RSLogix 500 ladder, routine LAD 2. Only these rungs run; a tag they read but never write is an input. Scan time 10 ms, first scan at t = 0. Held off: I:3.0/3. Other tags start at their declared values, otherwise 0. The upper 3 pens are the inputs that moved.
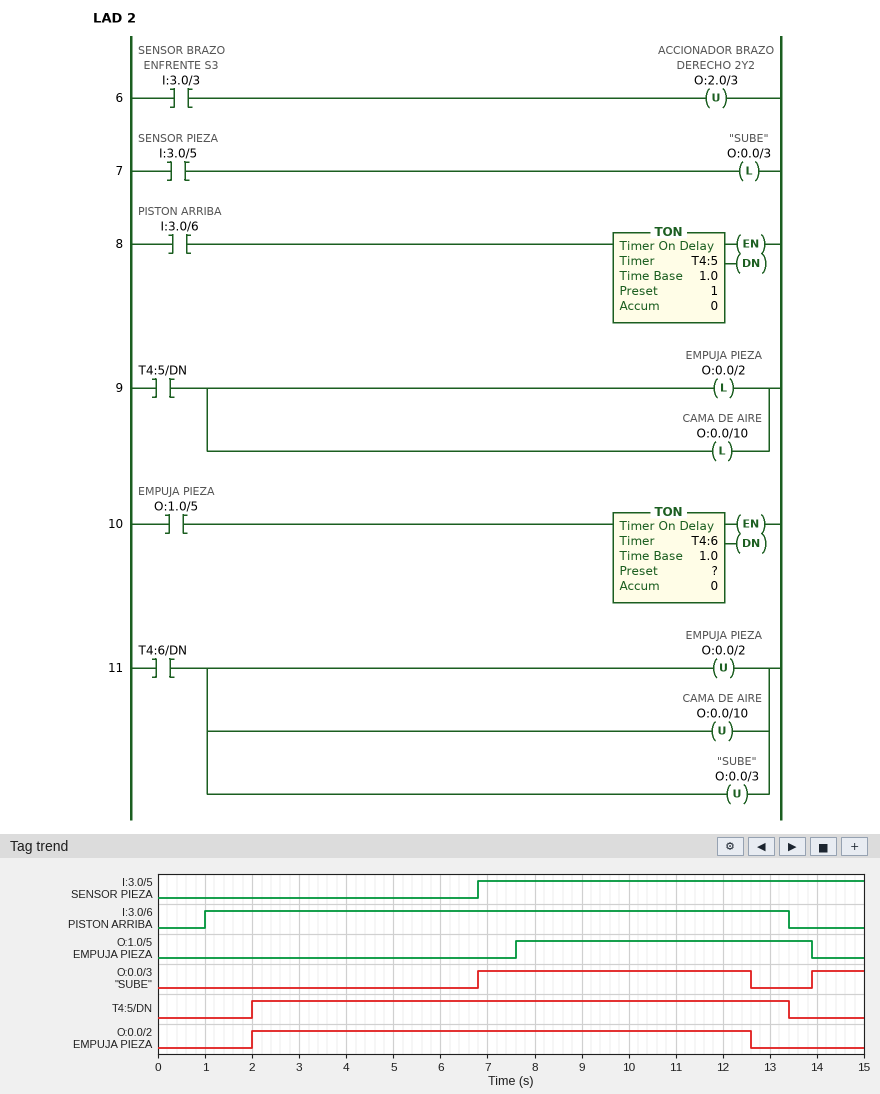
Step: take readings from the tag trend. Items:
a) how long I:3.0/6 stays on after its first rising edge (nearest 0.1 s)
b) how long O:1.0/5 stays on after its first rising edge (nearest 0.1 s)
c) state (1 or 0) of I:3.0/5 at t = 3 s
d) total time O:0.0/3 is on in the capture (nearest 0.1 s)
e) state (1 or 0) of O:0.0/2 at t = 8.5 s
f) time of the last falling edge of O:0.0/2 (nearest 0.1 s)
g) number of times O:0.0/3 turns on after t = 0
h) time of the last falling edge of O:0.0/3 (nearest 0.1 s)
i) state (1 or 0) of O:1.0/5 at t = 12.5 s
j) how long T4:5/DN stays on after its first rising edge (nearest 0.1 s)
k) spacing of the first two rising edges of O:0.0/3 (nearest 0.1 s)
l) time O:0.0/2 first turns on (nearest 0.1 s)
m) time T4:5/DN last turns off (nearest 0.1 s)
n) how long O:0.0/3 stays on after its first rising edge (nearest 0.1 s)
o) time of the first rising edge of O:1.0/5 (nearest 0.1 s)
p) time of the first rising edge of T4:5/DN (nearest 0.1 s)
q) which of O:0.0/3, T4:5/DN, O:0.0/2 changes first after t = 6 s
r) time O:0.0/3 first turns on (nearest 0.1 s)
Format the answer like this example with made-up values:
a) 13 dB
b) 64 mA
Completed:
a) 12.4 s
b) 6.3 s
c) 0
d) 6.9 s
e) 1
f) 12.6 s
g) 2
h) 12.6 s
i) 1
j) 11.4 s
k) 7.1 s
l) 2.0 s
m) 13.4 s
n) 5.8 s
o) 7.6 s
p) 2.0 s
q) O:0.0/3
r) 6.8 s
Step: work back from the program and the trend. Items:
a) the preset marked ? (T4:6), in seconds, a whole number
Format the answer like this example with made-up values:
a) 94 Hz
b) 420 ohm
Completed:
a) 5 s
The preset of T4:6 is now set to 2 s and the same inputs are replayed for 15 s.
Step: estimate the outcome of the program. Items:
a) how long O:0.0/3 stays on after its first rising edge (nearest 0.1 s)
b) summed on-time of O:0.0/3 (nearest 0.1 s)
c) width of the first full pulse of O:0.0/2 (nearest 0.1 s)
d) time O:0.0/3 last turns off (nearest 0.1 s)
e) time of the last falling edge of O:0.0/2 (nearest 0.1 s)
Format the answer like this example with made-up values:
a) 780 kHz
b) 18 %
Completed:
a) 2.8 s
b) 3.9 s
c) 7.6 s
d) 9.6 s
e) 9.6 s
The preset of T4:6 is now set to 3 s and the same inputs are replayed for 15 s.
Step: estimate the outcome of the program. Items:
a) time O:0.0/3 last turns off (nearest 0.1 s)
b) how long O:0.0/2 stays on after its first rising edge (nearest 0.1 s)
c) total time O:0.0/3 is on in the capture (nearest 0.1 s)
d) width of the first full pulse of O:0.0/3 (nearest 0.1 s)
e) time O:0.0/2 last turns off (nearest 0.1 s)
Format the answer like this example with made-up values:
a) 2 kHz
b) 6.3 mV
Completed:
a) 10.6 s
b) 8.6 s
c) 4.9 s
d) 3.8 s
e) 10.6 s
